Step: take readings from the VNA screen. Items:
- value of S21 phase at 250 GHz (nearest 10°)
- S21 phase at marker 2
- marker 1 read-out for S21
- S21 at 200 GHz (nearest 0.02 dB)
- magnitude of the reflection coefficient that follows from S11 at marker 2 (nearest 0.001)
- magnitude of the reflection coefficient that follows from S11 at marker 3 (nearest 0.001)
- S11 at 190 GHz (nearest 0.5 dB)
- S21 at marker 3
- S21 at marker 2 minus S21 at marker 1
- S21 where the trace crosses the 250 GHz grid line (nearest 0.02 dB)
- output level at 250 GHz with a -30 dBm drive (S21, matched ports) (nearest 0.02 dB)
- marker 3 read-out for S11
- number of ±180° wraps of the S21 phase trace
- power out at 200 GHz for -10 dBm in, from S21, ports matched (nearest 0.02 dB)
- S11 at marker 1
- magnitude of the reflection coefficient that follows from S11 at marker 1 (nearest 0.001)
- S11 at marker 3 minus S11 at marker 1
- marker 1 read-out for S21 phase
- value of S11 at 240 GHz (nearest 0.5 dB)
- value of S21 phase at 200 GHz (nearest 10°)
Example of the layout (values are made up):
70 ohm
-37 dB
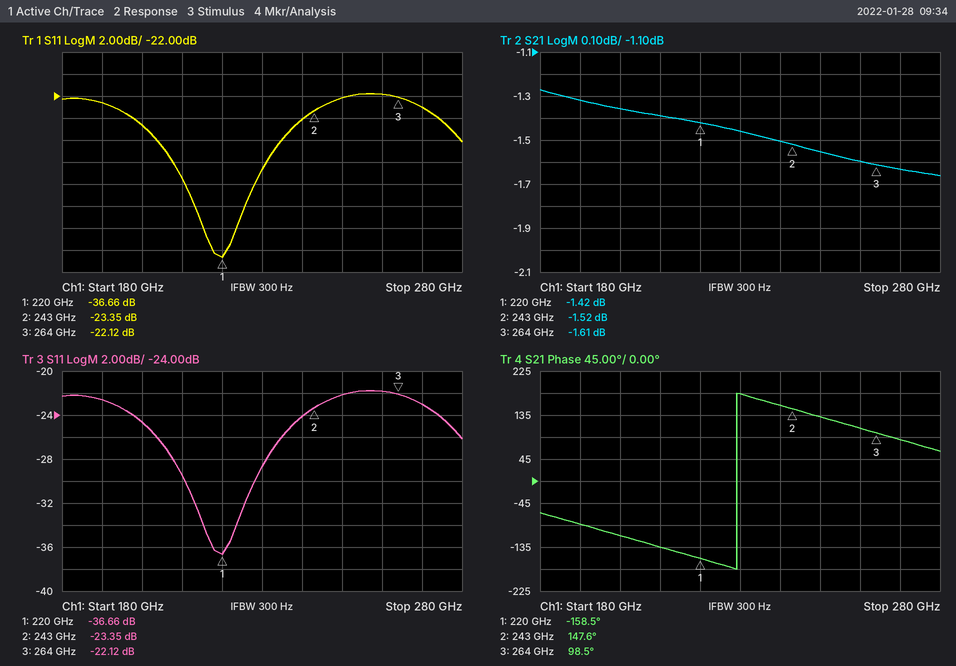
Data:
130°
147.6°
-1.42 dB
-1.36 dB
0.068
0.078
-22.5 dB
-1.61 dB
-0.10 dB
-1.56 dB
-31.56 dBm
-22.12 dB
1
-11.36 dBm
-36.66 dB
0.015
14.54 dB
-158.5°
-24.0 dB
-110°
